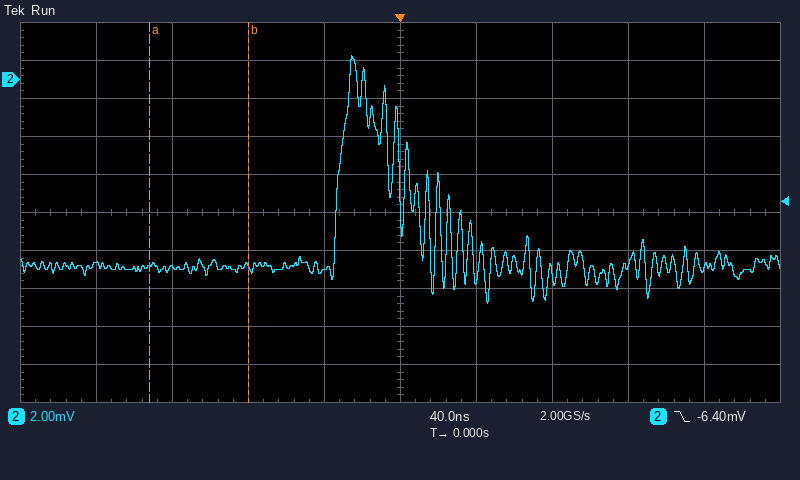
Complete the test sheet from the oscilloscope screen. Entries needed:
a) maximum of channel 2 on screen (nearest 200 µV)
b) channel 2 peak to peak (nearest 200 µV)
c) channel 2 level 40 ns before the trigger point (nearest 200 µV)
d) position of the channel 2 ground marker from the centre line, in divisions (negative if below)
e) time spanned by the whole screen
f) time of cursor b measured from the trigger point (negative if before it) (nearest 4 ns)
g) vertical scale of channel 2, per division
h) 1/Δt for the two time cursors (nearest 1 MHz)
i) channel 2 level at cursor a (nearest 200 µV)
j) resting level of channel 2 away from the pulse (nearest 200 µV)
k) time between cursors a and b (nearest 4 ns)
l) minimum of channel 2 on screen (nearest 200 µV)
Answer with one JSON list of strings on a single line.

["1.2 mV", "13.0 mV", "-10.0 mV", "+3.5 div", "400 ns", "-80 ns", "2 mV", "19 MHz", "-9.8 mV", "-9.8 mV", "52 ns", "-11.8 mV"]
